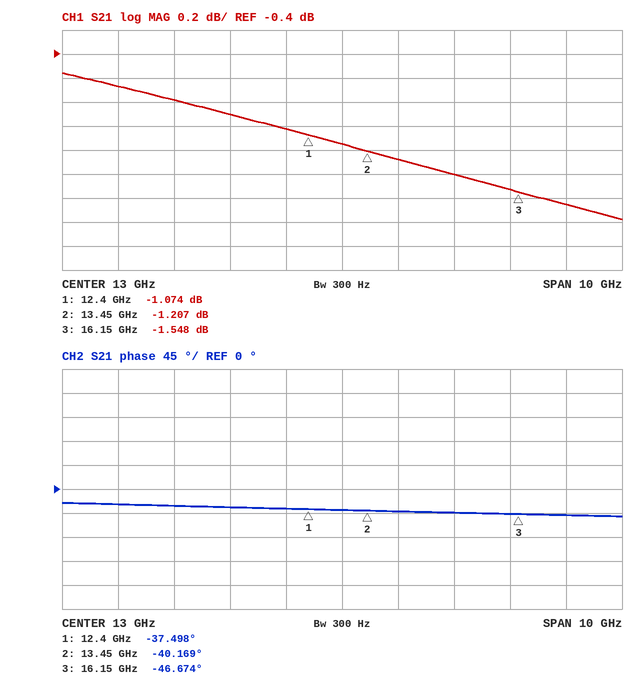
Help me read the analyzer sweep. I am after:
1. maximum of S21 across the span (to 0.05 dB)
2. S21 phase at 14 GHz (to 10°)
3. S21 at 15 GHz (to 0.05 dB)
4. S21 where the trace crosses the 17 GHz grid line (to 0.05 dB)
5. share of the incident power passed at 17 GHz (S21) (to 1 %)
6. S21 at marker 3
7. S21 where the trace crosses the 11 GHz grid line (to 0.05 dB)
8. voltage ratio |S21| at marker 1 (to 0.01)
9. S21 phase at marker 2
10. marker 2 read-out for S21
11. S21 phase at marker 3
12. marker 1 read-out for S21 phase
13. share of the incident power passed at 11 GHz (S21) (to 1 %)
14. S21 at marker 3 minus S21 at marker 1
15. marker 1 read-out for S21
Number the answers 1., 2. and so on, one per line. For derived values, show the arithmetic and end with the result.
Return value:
1. -0.55 dB
2. -40°
3. -1.40 dB
4. -1.65 dB
5. 10^(-1.65/10) ≈ 68 %
6. -1.548 dB
7. -0.90 dB
8. 10^(-1.074/20) ≈ 0.88
9. -40.169°
10. -1.207 dB
11. -46.674°
12. -37.498°
13. 10^(-0.9/10) ≈ 81 %
14. -1.548 − (-1.074) = -0.474 dB
15. -1.074 dB
